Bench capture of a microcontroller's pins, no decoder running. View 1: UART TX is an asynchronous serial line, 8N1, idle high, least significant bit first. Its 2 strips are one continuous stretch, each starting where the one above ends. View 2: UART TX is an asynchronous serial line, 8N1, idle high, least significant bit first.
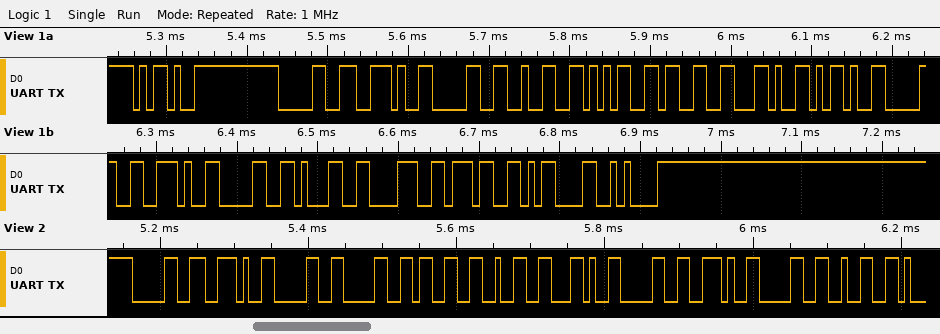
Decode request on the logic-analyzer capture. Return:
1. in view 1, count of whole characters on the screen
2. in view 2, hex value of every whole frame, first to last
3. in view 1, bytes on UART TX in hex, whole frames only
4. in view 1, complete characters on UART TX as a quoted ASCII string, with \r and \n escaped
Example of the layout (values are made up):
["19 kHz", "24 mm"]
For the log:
["17", "30 2E 30 30 33 32 2C 30 2E 30 32", "2D 30 2E 30 32 35 33 2C 2D 30 2E 30 31 38 37 0D 0A", "\"-0.0253,-0.0187\\r\\n\""]
